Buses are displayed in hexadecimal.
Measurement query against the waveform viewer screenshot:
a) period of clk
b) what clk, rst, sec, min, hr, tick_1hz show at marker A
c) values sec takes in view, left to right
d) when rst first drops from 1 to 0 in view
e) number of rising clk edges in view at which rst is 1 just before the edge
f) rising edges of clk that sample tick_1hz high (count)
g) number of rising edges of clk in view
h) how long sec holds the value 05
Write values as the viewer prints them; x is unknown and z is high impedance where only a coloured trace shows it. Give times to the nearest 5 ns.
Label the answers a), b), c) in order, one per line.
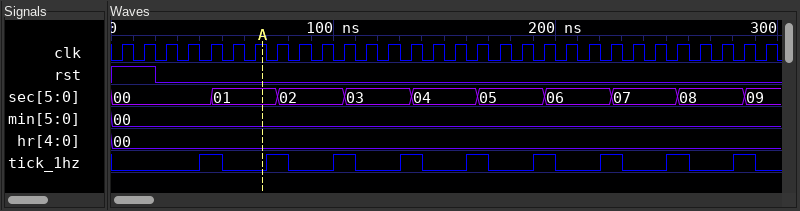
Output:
a) 10 ns
b) clk=1, rst=0, sec=01, min=00, hr=00, tick_1hz=0
c) 00, 01, 02, 03, 04, 05, 06, 07, 08, 09
d) 20 ns
e) 2
f) 9
g) 30
h) 30 ns
